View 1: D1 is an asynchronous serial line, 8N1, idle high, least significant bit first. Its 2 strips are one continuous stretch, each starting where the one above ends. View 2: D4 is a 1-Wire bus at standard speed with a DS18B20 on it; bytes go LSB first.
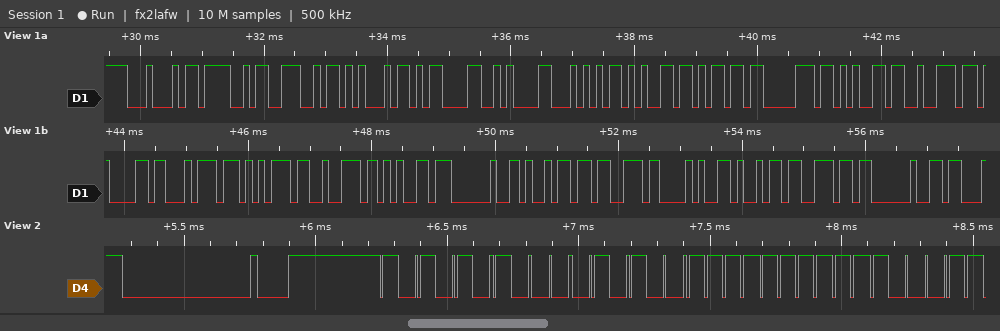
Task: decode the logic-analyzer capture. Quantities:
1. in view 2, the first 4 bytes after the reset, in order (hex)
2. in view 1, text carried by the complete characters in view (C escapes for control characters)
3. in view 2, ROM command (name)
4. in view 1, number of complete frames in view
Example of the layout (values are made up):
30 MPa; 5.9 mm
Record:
55 28 FF C7; "DONE\r\nTemperature is(in "; Match ROM; 24
